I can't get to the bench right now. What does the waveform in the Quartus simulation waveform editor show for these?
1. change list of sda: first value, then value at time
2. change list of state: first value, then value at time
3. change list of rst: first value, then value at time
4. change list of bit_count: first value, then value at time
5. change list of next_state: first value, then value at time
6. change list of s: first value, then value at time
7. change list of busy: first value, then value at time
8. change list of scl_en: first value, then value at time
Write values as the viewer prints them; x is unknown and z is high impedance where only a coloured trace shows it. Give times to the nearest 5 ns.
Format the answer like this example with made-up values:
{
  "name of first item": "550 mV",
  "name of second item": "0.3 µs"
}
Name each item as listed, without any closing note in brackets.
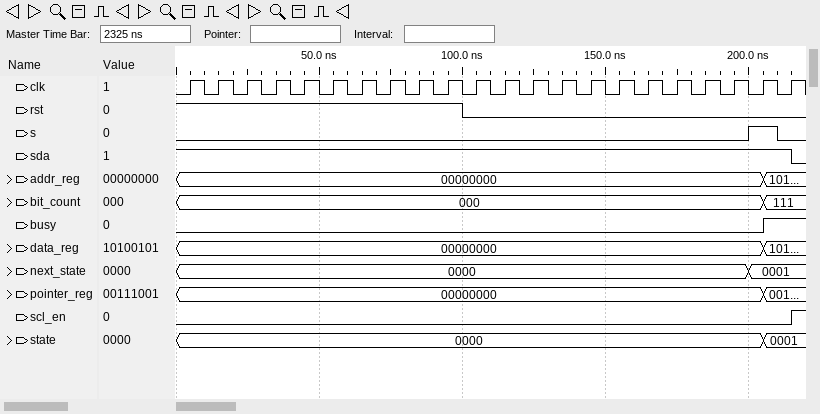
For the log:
{
  "change list of sda: first value, then value at time": "1, 0 at 215 ns",
  "change list of state: first value, then value at time": "0000, 0001 at 205 ns",
  "change list of rst: first value, then value at time": "1, 0 at 100 ns",
  "change list of bit_count: first value, then value at time": "000, 111 at 205 ns",
  "change list of next_state: first value, then value at time": "0000, 0001 at 200 ns",
  "change list of s: first value, then value at time": "0, 1 at 200 ns, 0 at 210 ns",
  "change list of busy: first value, then value at time": "0, 1 at 205 ns",
  "change list of scl_en: first value, then value at time": "0, 1 at 215 ns"
}
